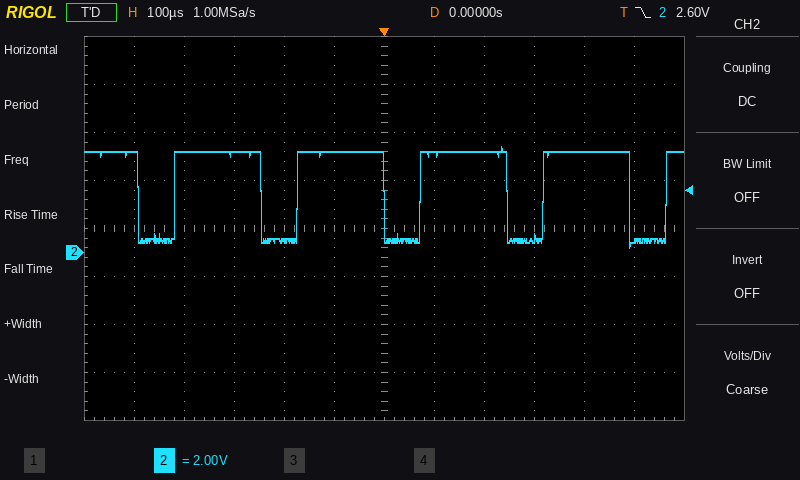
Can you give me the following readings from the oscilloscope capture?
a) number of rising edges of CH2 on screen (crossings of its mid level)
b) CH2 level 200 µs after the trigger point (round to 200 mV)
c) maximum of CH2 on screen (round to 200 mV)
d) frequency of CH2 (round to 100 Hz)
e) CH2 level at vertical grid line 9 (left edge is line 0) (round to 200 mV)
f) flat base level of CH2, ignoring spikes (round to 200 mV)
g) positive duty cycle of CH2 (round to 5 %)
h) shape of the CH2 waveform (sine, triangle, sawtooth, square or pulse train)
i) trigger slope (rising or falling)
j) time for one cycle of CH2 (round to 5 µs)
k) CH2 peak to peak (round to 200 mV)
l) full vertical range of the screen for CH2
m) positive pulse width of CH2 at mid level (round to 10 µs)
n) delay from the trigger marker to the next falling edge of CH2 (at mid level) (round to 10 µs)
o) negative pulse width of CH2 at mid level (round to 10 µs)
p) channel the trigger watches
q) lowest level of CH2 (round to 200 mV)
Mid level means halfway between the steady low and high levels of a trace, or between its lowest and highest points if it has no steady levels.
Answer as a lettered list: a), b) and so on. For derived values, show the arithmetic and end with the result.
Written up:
a) 5
b) 4.2 V
c) 4.4 V
d) 1 / 245 µs ≈ 4.1 kHz
e) 600 mV
f) 600 mV
g) 170 µs / 245 µs ≈ 69.4 %, so 70 % to the nearest 5 %
h) pulse train
i) falling
j) 245 µs
k) 4.4 V − (200 mV) = 4.2 V
l) 16 V
m) 170 µs
n) 250 µs
o) 70 µs
p) CH2
q) 200 mV
